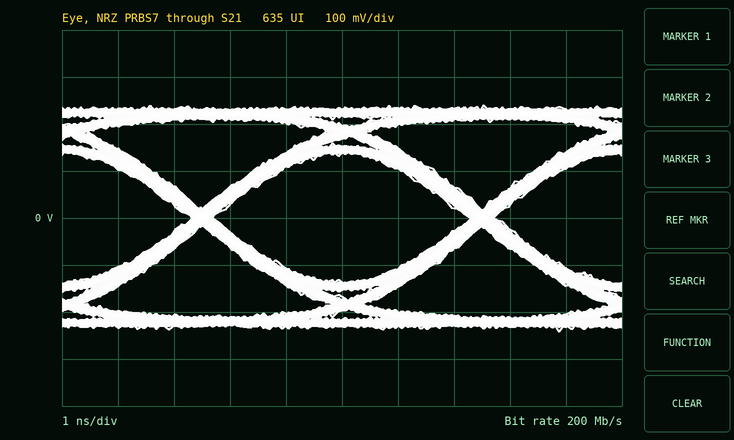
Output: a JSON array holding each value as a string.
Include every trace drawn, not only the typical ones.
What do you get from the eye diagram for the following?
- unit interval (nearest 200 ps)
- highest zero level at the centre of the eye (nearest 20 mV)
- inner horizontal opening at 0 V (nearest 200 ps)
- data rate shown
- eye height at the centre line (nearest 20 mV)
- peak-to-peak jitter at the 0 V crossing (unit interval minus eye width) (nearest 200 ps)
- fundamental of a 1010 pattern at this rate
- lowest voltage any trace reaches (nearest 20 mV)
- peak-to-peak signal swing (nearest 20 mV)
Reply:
["5.0 ns", "-140 mV", "4.6 ns", "200 Mb/s", "280 mV", "400 ps", "100 MHz", "-240 mV", "480 mV"]
